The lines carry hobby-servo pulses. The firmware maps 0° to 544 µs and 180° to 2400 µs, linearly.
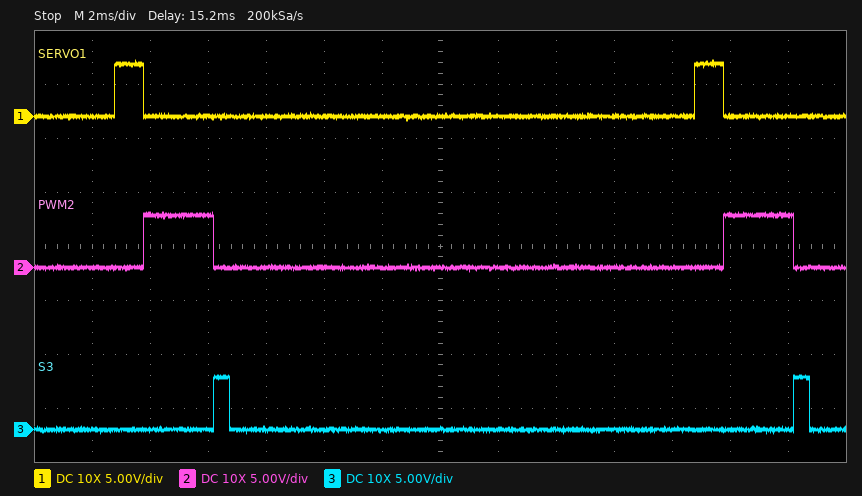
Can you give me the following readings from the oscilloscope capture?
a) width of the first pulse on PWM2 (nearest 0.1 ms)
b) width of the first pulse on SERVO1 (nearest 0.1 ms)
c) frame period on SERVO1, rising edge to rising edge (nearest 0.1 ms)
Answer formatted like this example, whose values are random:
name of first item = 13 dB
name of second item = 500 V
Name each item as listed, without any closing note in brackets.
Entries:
width of the first pulse on PWM2 = 2.4 ms
width of the first pulse on SERVO1 = 1.0 ms
frame period on SERVO1, rising edge to rising edge = 20.0 ms
